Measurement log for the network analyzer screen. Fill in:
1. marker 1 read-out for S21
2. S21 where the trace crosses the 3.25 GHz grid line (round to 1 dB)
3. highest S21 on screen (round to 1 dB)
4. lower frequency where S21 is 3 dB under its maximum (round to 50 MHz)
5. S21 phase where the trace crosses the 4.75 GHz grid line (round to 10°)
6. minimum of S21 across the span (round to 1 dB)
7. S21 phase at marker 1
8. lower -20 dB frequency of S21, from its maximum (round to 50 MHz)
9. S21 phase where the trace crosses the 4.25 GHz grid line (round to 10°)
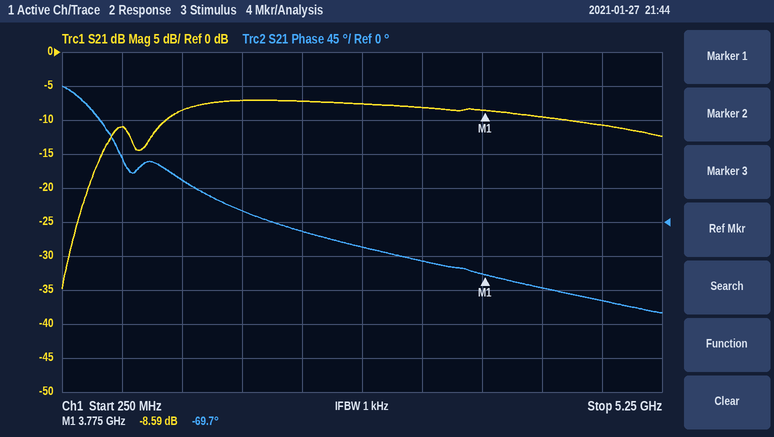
-8.59 dB
-8 dB
-7 dB
1.10 GHz
-100°
-35 dB
-69.7°
350 MHz
-90°
